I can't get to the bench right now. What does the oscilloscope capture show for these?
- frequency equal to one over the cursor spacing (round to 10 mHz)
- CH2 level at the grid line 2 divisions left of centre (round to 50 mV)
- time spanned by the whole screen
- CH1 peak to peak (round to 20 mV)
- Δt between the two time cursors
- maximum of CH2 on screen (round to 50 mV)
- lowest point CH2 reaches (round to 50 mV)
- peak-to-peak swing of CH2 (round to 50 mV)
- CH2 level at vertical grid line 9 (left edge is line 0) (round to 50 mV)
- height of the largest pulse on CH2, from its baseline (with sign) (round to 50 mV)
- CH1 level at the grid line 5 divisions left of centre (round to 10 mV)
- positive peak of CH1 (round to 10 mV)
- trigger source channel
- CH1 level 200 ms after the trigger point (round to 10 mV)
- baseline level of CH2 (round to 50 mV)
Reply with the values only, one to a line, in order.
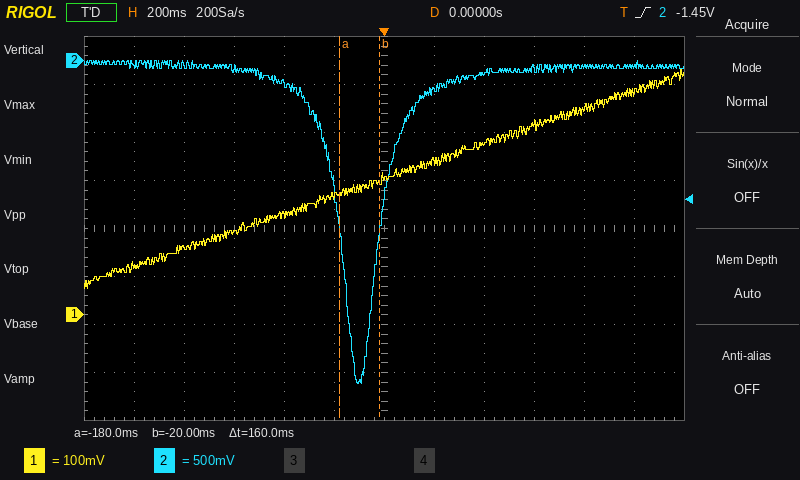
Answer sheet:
6.25 Hz
-250 mV
2.4 s
460 mV
160 ms
0 mV
-3.35 V
3.35 V
-100 mV
-3.30 V
100 mV
510 mV
CH2
320 mV
-50 mV
